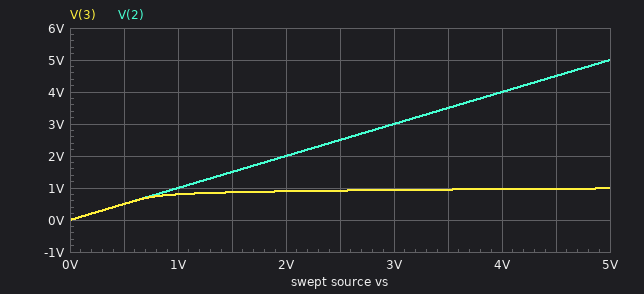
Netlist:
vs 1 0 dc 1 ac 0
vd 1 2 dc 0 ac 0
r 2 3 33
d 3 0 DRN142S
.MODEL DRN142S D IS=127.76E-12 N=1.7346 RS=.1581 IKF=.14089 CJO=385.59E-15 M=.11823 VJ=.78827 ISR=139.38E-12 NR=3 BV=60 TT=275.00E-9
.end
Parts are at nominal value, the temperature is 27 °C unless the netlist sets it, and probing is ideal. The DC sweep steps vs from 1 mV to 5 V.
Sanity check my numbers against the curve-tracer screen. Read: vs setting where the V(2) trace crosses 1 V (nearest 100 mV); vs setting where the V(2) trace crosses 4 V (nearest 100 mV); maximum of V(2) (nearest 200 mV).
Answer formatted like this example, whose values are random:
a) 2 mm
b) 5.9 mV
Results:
a) 1.0 V
b) 4.0 V
c) 5.0 V
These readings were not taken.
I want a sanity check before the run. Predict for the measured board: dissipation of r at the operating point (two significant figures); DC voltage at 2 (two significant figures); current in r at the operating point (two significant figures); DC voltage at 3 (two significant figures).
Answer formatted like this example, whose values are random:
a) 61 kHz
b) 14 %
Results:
a) 1.2 mW
b) 1.0 V
c) 6.0 mA
d) 800 mV
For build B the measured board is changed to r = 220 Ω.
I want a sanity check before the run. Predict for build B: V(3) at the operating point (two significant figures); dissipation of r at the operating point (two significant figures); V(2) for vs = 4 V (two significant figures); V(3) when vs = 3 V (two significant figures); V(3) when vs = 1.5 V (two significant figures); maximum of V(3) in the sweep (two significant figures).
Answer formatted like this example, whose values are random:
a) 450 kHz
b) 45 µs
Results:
a) 730 mV
b) 340 µW
c) 4.0 V
d) 830 mV
e) 770 mV
f) 860 mV
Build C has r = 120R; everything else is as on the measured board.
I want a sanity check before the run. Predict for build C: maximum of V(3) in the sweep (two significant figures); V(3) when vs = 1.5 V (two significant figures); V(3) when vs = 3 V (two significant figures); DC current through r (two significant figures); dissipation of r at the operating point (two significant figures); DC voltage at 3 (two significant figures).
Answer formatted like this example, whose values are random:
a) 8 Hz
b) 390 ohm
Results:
a) 900 mV
b) 800 mV
c) 860 mV
d) 2.1 mA
e) 520 µW
f) 750 mV
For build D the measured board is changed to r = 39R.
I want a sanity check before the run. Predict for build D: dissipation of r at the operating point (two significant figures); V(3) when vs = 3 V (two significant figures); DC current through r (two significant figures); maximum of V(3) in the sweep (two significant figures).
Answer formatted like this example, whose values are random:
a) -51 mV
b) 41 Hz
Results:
a) 1.1 mW
b) 930 mV
c) 5.2 mA
d) 970 mV
